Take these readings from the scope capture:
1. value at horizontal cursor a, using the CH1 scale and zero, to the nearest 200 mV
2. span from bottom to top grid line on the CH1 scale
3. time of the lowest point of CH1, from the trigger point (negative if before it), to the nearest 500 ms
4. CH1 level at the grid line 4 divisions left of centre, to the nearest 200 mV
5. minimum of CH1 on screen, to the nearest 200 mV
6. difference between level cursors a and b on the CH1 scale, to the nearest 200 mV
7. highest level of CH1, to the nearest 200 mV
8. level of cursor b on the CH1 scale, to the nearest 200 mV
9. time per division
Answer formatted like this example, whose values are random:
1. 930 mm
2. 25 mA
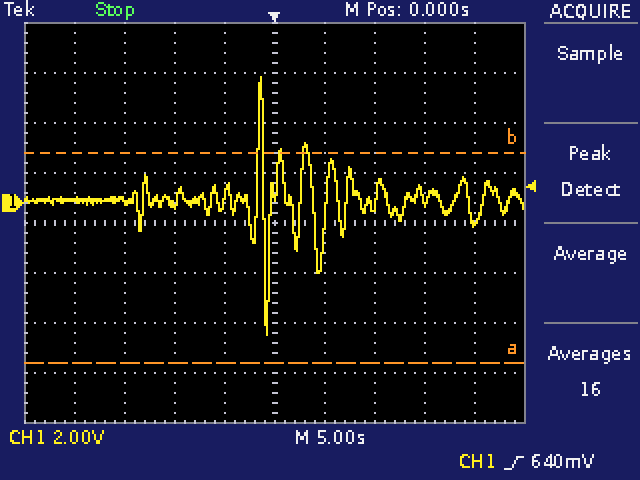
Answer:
1. -6.4 V
2. 16 V
3. -500 ms
4. 200 mV
5. -5.2 V
6. 8.4 V
7. 5.0 V
8. 2.0 V
9. 5 s
